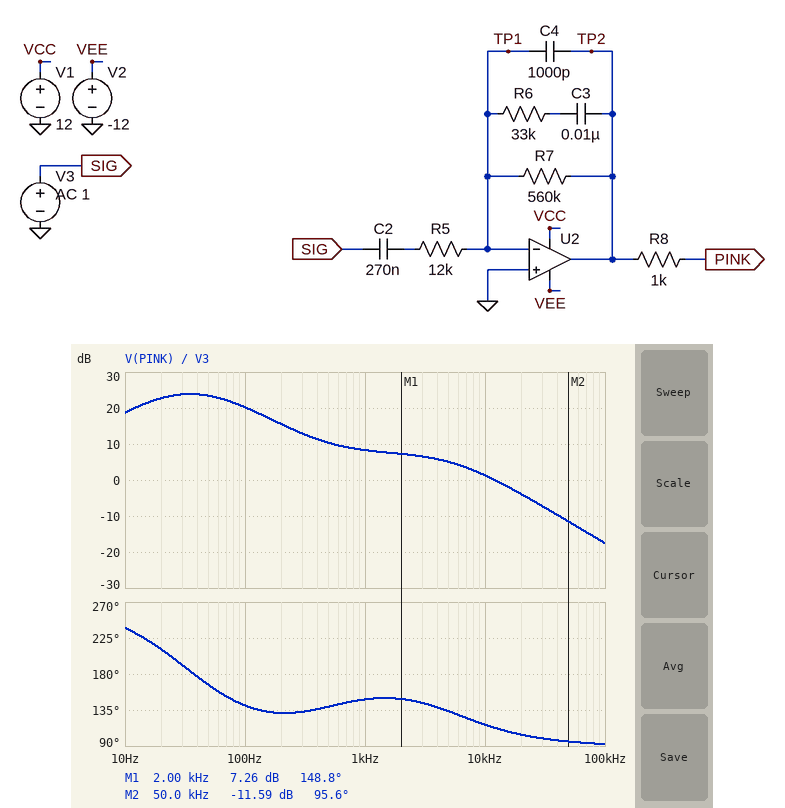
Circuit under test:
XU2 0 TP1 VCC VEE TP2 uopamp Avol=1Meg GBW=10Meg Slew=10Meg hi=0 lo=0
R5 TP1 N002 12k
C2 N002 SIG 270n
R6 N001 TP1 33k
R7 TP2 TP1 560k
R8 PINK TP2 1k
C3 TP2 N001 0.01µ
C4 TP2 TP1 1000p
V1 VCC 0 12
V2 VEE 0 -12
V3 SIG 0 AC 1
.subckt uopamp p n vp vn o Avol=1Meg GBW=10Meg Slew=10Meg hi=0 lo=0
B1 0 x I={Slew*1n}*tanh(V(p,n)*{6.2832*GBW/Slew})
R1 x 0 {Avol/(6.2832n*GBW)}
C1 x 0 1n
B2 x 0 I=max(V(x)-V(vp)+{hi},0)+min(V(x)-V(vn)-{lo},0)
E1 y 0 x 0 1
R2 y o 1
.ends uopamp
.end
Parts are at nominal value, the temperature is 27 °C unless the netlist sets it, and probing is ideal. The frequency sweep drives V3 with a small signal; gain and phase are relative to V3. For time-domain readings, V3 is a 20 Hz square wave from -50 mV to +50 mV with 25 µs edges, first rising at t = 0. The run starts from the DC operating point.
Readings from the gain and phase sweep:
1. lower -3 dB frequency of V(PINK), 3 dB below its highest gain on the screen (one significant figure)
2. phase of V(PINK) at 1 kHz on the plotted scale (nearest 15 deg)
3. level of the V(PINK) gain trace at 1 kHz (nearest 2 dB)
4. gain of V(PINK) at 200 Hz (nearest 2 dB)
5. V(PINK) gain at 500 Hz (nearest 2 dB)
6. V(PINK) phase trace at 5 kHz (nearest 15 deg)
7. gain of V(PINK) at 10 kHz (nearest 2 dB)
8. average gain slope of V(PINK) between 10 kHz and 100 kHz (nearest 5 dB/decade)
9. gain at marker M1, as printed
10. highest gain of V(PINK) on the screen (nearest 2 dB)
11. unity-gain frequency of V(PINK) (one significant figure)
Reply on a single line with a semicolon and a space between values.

10 Hz; 150 deg; 8 dB; 16 dB; 10 dB; 135 deg; 2 dB; -20 dB/decade; 7.26 dB; 24 dB; 10 kHz
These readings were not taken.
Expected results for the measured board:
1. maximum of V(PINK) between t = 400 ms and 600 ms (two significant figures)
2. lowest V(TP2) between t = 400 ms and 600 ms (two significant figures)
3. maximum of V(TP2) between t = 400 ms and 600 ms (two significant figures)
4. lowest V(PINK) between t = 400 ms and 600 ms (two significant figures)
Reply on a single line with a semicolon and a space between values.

1.1 V; -1.1 V; 1.1 V; -1.1 V
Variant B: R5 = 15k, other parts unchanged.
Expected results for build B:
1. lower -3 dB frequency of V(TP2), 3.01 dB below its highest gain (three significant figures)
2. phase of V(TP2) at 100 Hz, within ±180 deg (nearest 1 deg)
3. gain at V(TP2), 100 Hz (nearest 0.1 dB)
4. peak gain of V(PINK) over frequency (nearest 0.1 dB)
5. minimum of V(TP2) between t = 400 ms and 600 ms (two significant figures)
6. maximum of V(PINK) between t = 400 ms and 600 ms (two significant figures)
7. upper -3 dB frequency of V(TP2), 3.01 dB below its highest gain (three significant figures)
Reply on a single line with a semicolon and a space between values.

12.7 Hz; 136 deg; 18.6 dB; 23.2 dB; -1.0 V; 1.0 V; 77.7 Hz
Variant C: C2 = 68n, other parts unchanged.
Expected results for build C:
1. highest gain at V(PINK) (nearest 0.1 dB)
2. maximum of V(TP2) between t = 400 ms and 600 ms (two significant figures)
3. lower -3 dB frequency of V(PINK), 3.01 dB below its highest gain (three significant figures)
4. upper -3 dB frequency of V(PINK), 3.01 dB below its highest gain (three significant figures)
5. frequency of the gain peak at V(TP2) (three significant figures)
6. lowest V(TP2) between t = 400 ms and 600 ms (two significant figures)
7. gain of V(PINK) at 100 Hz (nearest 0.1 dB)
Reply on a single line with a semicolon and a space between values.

14.5 dB; 430 mV; 20.4 Hz; 305 Hz; 73.3 Hz; -430 mV; 14.3 dB
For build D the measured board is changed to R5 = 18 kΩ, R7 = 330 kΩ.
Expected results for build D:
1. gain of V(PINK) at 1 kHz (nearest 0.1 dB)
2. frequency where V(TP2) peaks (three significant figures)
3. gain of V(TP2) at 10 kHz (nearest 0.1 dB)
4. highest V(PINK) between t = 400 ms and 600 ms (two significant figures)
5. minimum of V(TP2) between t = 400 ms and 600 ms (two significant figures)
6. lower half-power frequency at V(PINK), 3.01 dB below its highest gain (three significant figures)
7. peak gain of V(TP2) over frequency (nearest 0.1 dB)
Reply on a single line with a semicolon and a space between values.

4.5 dB; 36.6 Hz; -2.3 dB; 730 mV; -730 mV; 15.1 Hz; 20.1 dB
